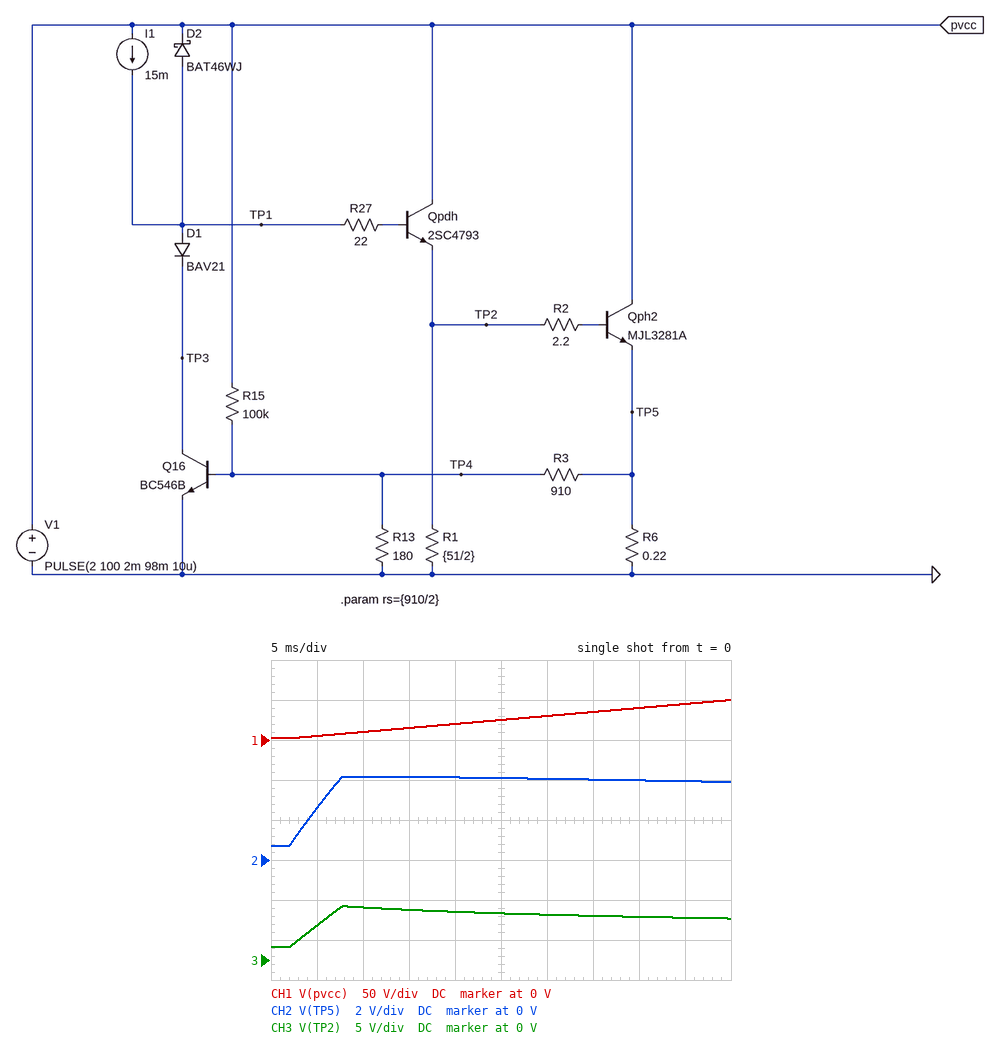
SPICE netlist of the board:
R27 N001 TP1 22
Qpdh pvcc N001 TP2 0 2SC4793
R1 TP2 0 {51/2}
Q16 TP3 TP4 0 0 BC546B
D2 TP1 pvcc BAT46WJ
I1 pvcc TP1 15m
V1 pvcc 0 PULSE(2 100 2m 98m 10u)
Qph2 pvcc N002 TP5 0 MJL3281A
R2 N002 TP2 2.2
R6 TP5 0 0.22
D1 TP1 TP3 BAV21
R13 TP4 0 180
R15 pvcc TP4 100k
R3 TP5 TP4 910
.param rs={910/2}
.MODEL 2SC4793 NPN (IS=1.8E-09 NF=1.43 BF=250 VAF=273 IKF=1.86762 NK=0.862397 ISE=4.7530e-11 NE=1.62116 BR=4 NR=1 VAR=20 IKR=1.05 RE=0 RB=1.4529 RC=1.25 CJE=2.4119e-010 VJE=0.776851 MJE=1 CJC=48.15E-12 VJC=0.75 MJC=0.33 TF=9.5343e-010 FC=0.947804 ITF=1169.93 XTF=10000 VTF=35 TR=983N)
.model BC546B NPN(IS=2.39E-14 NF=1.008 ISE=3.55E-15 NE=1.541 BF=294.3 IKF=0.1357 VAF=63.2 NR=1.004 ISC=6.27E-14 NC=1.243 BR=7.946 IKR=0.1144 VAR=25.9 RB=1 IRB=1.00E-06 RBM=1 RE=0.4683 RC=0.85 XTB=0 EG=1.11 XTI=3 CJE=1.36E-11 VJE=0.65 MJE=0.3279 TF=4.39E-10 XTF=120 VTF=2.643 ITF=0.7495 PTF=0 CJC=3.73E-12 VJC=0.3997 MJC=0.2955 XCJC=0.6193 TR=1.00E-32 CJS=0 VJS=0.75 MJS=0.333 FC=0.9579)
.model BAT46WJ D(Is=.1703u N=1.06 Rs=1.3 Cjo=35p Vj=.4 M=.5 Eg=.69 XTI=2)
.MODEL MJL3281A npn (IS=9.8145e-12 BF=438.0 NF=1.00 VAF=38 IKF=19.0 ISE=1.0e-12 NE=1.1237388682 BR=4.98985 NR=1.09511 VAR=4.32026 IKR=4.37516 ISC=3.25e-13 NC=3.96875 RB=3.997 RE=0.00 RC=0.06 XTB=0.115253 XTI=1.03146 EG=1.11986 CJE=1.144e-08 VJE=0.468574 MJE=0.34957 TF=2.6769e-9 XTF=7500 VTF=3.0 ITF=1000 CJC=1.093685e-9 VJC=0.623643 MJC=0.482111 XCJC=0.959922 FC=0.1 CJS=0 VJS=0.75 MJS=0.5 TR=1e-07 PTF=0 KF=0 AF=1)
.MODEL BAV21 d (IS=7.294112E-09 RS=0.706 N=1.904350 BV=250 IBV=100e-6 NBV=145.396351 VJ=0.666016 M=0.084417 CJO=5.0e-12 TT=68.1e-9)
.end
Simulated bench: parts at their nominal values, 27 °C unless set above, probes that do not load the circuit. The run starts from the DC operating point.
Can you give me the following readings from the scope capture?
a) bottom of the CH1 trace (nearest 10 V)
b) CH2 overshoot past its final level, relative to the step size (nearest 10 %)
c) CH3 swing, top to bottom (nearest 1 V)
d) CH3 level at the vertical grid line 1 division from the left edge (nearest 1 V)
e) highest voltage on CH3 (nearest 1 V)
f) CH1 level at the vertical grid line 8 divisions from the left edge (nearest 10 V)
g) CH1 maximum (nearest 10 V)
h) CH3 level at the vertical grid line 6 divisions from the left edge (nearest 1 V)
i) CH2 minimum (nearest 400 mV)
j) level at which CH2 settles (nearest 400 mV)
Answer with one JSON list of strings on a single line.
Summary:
["0 V", "10 %", "5 V", "4 V", "7 V", "40 V", "50 V", "6 V", "800 mV", "4.0 V"]
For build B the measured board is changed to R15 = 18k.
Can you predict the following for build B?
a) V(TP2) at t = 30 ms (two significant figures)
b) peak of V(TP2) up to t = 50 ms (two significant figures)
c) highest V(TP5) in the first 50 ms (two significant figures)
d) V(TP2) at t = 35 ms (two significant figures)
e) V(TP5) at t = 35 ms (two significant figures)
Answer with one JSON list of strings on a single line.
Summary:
["4.1 V", "6.3 V", "3.9 V", "3.8 V", "2.6 V"]
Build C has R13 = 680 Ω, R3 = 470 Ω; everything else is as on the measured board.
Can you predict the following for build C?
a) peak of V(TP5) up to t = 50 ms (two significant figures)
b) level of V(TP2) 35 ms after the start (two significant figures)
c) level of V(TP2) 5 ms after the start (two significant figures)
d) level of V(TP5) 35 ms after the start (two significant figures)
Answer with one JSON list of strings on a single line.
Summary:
["1.2 V", "1.9 V", "2.3 V", "1.1 V"]
